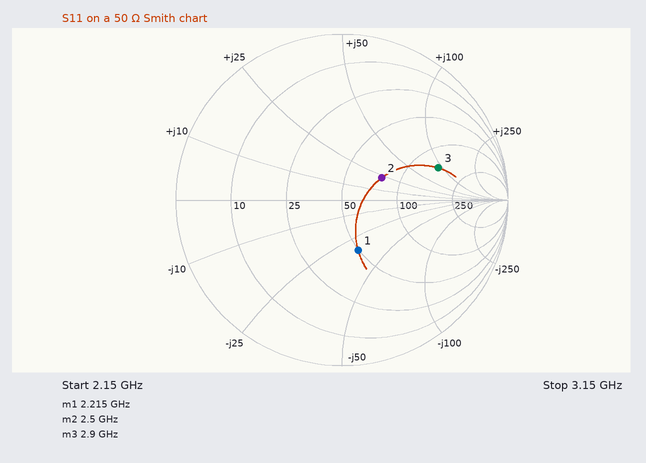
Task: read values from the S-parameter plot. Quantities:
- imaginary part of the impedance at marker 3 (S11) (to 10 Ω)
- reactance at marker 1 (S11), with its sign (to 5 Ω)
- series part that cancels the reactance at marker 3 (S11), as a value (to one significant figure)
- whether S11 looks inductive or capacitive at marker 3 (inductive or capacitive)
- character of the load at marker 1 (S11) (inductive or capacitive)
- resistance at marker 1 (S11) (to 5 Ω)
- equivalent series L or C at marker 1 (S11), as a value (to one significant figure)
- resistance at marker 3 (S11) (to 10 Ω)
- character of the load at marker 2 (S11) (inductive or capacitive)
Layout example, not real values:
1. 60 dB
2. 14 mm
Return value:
1. +90 Ω
2. -35 Ω
3. 600 fF
4. inductive
5. capacitive
6. 50 Ω
7. 2 pF
8. 150 Ω
9. inductive
